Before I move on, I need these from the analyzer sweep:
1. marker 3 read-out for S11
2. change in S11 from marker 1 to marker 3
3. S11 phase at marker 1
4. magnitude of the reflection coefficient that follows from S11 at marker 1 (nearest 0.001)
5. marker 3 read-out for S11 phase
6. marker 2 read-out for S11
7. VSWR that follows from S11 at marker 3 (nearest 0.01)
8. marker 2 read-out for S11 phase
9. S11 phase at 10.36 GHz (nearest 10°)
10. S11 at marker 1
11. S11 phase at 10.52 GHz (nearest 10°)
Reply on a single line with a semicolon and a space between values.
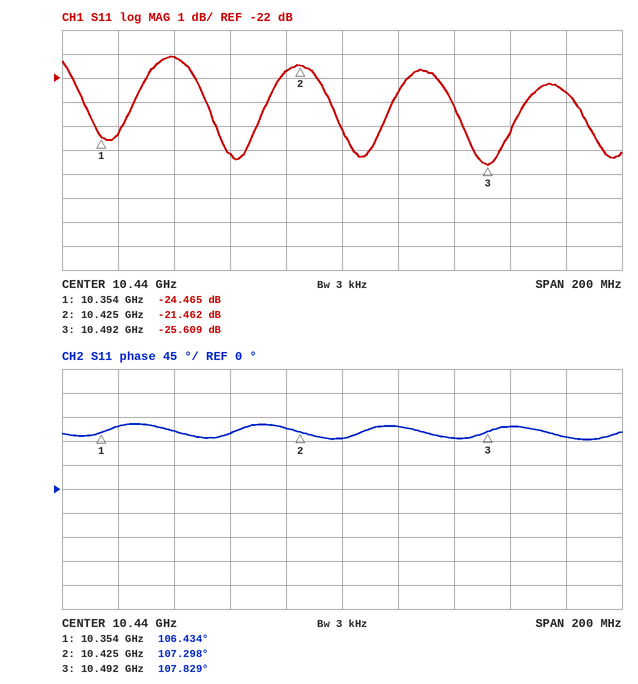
-25.609 dB; -1.144 dB; 106.434°; 0.060; 107.829°; -21.462 dB; 1.11; 107.298°; 120°; -24.465 dB; 100°
